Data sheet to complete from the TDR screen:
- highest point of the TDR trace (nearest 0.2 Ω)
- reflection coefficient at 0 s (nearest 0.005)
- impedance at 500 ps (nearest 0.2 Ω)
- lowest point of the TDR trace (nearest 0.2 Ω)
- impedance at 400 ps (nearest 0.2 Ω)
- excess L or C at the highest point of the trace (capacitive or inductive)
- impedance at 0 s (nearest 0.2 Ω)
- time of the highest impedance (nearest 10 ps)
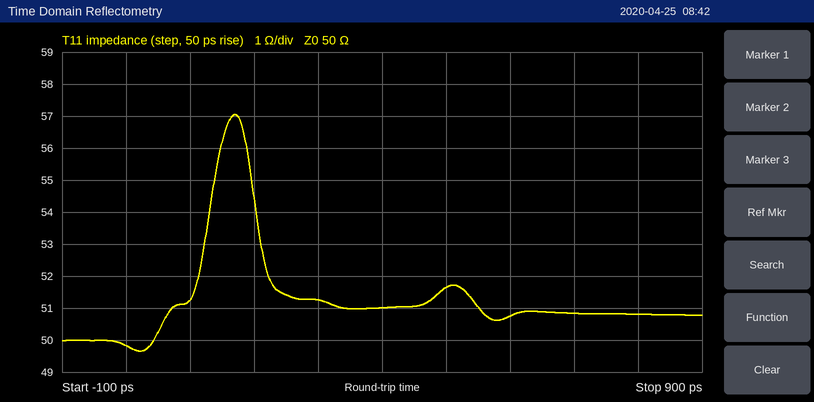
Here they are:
57.0 Ω
0.000
51.6 Ω
49.6 Ω
51.0 Ω
inductive
49.8 Ω
170 ps
